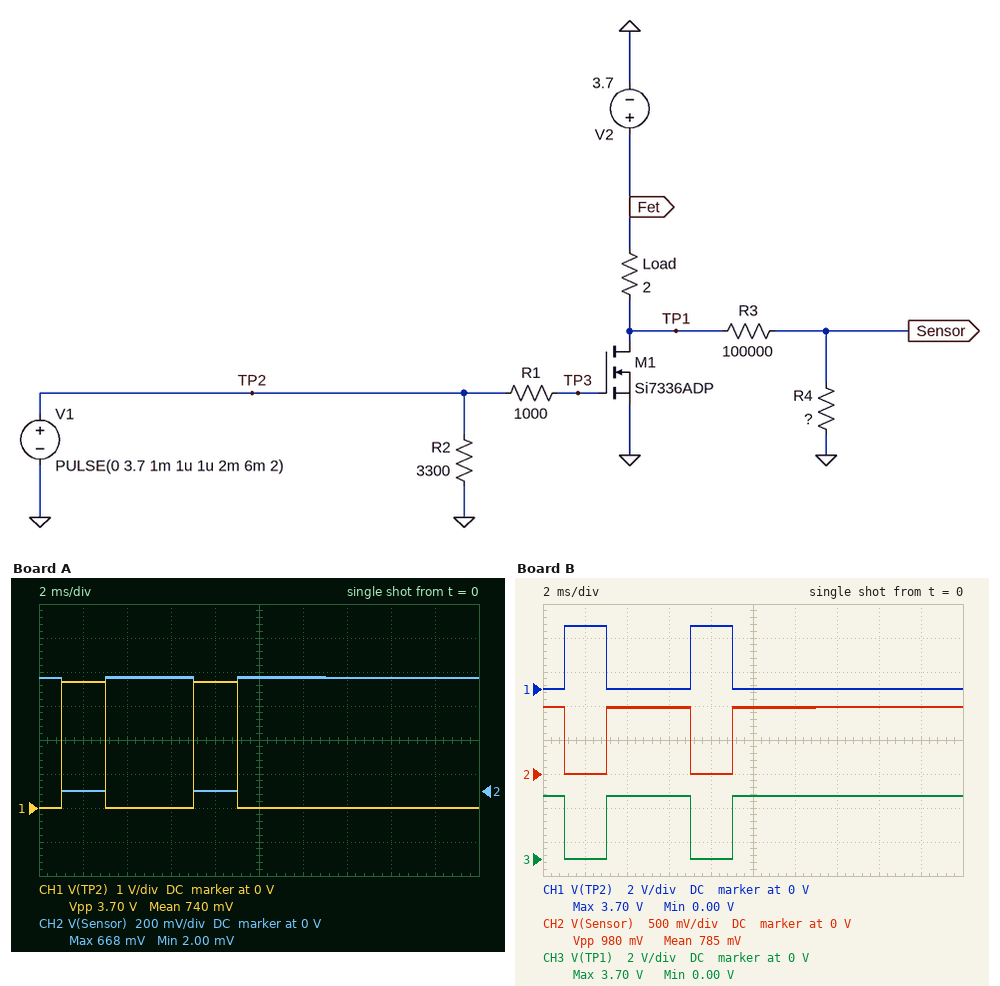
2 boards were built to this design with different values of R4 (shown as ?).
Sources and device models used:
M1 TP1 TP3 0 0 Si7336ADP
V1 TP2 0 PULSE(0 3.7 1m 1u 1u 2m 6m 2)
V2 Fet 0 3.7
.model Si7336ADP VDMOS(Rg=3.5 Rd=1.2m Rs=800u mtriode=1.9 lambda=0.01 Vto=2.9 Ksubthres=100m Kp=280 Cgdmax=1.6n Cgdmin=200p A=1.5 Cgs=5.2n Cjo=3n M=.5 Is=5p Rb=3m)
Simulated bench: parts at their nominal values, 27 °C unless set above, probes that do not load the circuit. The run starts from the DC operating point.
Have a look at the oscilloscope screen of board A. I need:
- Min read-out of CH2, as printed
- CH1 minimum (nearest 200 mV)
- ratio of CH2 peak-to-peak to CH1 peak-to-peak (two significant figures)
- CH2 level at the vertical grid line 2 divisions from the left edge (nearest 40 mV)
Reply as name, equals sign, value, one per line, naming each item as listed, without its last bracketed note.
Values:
Min read-out of CH2, as printed = 2.00 mV
CH1 minimum = 0 V
ratio of CH2 peak-to-peak to CH1 peak-to-peak = 0.18
CH2 level at the vertical grid line 2 divisions from the left edge = 680 mV
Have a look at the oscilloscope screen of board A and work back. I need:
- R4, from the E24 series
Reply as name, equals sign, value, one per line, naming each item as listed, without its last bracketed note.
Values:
R4, from the E24 series = 22 kΩ
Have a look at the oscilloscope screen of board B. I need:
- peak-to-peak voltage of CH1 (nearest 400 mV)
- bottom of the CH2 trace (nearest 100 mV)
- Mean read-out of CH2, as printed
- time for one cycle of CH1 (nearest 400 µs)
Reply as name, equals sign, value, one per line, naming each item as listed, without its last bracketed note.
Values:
peak-to-peak voltage of CH1 = 3.6 V
bottom of the CH2 trace = 0 V
Mean read-out of CH2, as printed = 785 mV
time for one cycle of CH1 = 6.0 ms
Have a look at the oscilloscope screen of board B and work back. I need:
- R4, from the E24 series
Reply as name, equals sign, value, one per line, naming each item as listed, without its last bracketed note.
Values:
R4, from the E24 series = 36 kΩ
